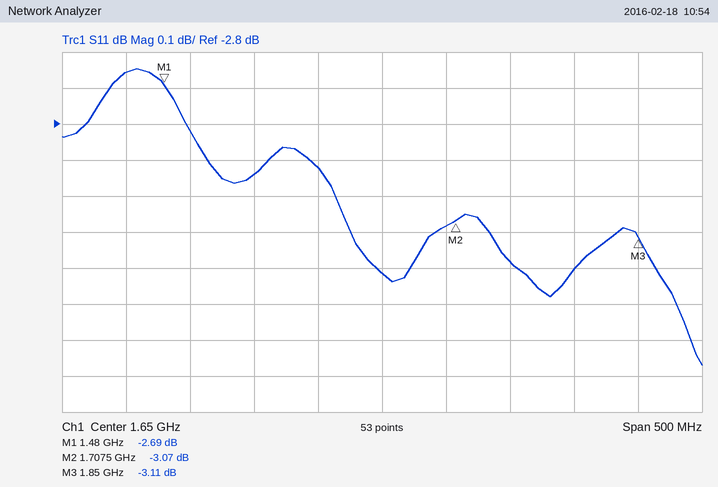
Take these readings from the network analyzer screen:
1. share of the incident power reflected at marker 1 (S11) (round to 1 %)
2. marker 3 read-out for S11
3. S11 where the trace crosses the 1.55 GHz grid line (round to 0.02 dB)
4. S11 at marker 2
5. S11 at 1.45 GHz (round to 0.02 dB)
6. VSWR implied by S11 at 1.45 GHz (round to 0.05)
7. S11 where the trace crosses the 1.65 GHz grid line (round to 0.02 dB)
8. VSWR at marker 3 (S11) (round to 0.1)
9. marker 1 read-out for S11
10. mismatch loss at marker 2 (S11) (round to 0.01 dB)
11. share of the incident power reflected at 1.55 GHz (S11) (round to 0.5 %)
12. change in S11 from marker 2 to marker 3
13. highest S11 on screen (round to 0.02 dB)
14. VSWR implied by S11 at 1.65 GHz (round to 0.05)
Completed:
54 %
-3.11 dB
-2.94 dB
-3.07 dB
-2.66 dB
6.60
-3.22 dB
5.6
-2.69 dB
2.95 dB
51.0 %
-0.04 dB
-2.64 dB
5.45
